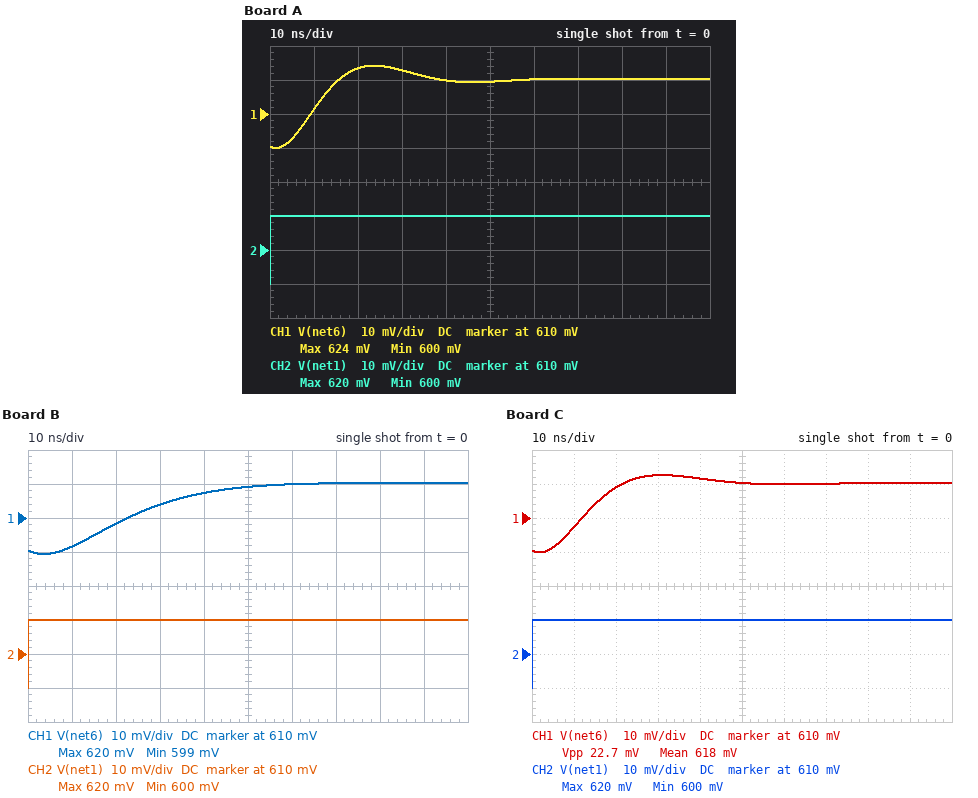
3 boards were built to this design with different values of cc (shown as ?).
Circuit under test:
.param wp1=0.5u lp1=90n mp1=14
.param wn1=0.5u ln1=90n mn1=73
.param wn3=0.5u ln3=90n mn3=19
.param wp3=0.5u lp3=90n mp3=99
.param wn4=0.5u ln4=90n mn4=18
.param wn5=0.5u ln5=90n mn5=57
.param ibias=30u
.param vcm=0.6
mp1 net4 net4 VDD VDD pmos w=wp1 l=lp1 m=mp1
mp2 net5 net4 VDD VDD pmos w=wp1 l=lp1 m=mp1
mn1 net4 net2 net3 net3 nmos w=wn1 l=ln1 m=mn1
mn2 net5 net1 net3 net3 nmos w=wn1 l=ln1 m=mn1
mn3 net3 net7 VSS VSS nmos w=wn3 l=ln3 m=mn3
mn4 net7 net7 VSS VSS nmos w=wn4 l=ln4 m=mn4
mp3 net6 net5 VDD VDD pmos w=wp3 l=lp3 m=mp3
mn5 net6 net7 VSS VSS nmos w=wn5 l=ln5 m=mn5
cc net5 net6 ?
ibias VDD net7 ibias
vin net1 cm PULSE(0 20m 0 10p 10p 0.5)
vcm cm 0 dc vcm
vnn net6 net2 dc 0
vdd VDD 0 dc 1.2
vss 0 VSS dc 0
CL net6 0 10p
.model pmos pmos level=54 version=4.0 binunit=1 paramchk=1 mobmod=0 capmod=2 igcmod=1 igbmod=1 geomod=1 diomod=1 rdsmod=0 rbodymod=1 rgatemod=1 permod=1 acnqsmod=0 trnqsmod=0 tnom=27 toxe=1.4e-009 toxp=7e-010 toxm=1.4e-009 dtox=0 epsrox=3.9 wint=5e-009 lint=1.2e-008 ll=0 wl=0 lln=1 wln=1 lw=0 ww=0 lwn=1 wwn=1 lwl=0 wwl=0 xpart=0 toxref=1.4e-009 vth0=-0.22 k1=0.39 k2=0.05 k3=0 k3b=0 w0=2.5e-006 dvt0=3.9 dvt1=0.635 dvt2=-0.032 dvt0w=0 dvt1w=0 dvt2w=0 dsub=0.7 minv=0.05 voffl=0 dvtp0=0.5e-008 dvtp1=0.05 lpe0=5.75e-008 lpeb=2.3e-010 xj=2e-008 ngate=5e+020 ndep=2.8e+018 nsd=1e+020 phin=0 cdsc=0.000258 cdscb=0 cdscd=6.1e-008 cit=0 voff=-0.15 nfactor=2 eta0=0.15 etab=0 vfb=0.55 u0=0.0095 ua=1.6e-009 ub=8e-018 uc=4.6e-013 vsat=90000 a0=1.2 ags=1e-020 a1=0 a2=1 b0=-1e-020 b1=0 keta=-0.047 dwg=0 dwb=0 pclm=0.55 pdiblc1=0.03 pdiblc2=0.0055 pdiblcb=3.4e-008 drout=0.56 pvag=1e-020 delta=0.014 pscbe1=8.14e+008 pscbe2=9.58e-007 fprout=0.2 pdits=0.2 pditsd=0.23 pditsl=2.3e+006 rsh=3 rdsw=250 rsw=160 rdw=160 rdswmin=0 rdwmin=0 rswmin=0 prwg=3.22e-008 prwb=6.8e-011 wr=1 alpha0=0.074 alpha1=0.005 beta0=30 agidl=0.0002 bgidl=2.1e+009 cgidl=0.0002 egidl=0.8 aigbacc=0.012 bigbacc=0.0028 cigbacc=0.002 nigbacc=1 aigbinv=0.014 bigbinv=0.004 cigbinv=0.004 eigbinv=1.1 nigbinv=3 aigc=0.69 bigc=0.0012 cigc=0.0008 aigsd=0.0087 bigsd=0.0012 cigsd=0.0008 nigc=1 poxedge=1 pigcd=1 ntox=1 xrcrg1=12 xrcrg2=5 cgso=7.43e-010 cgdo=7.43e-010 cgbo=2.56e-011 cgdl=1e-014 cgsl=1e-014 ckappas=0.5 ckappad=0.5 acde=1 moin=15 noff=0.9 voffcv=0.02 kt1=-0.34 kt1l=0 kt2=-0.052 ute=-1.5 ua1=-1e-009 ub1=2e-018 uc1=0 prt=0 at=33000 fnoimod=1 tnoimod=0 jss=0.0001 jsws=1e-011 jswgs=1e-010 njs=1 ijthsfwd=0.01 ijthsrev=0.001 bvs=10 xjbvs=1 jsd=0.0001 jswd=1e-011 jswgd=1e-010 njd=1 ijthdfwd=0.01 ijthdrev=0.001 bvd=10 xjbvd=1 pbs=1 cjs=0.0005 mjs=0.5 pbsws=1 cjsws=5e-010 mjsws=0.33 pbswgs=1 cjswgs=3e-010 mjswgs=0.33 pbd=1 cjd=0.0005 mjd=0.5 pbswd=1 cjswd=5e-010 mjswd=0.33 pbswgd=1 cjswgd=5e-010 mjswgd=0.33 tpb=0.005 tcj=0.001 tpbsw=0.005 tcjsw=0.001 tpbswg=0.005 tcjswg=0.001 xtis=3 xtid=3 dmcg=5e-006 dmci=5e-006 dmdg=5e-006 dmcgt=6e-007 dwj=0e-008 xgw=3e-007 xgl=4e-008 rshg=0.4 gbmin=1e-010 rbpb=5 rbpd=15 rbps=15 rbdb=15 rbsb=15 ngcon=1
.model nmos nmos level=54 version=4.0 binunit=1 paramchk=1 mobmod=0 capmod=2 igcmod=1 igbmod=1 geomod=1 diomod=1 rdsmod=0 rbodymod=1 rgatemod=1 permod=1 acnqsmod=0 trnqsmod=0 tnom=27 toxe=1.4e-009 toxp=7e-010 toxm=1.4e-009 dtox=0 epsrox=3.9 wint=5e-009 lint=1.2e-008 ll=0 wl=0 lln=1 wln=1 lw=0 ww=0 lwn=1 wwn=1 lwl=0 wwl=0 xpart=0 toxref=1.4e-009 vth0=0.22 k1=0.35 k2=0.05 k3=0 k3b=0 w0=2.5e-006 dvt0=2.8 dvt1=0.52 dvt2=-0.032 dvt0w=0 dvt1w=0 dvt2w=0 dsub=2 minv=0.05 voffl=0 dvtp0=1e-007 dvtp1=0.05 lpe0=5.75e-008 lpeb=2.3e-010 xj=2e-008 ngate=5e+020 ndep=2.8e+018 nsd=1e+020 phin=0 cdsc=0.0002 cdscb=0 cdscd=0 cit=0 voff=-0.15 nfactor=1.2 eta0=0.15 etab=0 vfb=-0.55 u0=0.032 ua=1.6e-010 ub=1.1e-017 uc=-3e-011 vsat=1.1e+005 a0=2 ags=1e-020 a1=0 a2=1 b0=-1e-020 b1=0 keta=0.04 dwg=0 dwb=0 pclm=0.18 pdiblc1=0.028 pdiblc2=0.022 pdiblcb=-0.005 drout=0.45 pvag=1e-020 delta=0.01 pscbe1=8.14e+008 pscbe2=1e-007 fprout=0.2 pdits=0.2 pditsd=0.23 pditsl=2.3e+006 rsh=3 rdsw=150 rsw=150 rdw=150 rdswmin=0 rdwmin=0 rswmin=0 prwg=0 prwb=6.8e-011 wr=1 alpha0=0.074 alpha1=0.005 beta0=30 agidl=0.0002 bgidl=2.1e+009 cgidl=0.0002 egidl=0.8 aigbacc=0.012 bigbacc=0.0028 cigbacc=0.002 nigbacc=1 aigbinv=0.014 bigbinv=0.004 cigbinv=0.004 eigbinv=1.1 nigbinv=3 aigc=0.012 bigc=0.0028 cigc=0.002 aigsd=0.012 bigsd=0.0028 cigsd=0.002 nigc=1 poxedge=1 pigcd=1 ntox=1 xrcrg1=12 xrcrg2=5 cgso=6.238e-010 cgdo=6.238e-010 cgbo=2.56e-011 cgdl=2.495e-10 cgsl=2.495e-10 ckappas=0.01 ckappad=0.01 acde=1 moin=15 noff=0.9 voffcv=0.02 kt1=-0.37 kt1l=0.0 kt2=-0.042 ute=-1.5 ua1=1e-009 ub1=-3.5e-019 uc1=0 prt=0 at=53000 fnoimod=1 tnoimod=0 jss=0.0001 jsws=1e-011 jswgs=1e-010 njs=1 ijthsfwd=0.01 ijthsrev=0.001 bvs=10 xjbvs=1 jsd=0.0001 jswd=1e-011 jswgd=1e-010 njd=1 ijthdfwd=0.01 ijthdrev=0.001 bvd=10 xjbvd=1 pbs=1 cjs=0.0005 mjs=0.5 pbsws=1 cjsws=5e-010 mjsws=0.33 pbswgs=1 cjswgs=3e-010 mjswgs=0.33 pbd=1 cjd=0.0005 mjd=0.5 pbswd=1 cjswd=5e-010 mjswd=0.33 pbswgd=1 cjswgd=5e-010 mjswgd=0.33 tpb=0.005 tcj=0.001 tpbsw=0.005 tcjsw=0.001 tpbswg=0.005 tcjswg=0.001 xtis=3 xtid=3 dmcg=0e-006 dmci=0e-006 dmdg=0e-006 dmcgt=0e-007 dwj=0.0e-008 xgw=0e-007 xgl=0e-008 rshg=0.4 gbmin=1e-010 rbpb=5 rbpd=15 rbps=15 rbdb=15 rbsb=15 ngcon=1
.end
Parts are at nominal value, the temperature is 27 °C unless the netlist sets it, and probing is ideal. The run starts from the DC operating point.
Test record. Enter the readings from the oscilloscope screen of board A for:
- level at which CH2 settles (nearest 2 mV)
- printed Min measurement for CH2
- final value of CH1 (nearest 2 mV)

620 mV
600 mV
620 mV
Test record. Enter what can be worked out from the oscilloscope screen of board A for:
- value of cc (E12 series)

2.2 pF
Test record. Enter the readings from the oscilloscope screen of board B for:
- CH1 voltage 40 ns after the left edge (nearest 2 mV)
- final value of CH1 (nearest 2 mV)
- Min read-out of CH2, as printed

618 mV
620 mV
600 mV
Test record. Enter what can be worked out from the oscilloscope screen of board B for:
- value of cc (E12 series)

8.2 pF
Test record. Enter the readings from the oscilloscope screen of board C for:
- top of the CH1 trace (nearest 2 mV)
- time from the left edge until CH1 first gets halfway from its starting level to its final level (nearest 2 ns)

622 mV
12 ns
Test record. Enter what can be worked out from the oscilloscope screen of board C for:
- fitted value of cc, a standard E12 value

3.3 pF
